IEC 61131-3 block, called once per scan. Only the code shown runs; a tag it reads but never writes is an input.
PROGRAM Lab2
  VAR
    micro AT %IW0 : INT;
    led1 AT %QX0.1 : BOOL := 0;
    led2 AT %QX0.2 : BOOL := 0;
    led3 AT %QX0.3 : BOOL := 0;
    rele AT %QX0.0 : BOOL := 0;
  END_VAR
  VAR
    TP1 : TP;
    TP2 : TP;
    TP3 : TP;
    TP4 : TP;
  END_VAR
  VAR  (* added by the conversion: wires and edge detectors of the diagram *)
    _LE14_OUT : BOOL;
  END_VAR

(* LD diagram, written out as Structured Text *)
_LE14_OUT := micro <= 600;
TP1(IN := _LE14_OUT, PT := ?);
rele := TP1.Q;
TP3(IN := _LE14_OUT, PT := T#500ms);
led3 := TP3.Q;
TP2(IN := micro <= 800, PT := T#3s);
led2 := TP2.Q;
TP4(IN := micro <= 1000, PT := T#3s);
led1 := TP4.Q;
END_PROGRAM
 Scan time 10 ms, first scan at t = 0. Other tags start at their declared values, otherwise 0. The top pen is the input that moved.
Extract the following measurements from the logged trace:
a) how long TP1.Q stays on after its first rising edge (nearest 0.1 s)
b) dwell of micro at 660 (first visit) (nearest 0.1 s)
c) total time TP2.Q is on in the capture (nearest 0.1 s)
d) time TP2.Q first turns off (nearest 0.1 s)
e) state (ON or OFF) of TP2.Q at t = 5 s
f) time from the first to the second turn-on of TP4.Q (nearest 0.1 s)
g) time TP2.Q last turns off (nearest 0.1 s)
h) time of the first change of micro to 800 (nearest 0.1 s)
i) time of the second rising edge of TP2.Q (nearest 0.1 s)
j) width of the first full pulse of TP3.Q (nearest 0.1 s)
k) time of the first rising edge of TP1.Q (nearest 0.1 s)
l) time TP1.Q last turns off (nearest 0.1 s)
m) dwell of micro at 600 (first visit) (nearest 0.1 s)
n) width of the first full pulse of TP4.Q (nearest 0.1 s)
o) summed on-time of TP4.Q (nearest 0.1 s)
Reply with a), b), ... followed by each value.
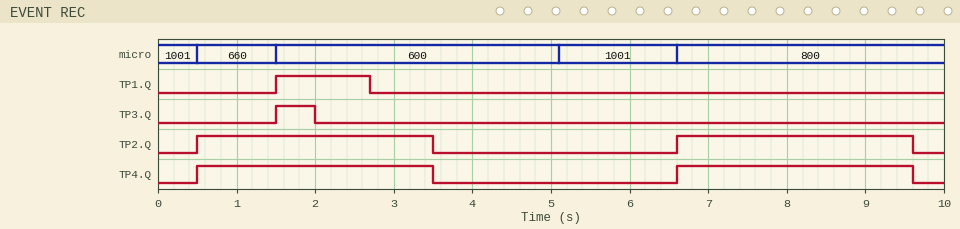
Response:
a) 1.2 s
b) 1.0 s
c) 6.0 s
d) 3.5 s
e) OFF
f) 6.1 s
g) 9.6 s
h) 6.6 s
i) 6.6 s
j) 0.5 s
k) 1.5 s
l) 2.7 s
m) 3.6 s
n) 3.0 s
o) 6.0 s
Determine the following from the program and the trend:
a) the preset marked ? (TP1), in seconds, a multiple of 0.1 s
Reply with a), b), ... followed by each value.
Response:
a) 1.2 s
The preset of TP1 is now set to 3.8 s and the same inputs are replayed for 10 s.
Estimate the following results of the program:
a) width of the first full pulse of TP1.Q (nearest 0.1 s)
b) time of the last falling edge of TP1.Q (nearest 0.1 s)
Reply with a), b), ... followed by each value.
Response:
a) 3.8 s
b) 5.3 s
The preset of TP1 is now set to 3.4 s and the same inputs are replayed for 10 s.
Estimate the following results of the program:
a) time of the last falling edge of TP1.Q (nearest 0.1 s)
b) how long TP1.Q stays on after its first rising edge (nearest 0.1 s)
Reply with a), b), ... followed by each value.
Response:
a) 4.9 s
b) 3.4 s
